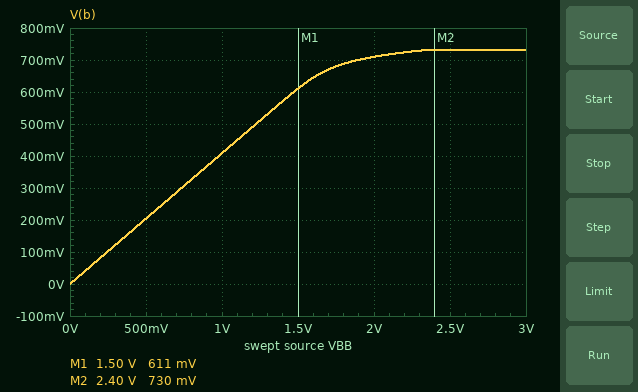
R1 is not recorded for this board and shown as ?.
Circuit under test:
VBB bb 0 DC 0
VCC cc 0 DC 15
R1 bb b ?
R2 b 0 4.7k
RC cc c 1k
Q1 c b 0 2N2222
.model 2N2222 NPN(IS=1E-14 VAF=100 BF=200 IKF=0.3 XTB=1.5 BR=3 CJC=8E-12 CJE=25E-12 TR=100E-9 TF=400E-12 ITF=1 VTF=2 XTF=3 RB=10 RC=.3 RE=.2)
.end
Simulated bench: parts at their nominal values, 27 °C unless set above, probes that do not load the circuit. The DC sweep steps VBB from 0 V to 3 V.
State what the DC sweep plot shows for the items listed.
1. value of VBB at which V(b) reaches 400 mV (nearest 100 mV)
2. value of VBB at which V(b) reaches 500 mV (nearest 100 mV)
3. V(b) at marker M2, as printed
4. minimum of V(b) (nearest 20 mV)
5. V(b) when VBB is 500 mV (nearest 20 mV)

1.0 V
1.2 V
730 mV
0 V
200 mV
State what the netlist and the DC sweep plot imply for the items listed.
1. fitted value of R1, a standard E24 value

6.8 kΩ
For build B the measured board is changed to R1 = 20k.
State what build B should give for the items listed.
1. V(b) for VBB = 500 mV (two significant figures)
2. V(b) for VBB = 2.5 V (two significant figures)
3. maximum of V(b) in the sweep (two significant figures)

95 mV
480 mV
570 mV
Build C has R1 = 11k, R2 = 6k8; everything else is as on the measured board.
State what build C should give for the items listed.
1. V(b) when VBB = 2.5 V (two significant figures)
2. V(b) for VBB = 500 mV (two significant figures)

720 mV
190 mV
